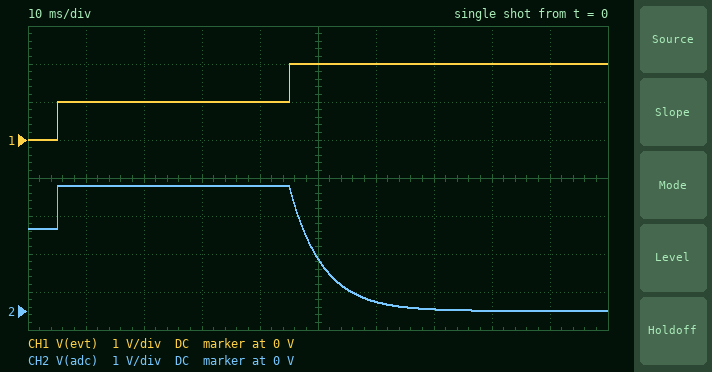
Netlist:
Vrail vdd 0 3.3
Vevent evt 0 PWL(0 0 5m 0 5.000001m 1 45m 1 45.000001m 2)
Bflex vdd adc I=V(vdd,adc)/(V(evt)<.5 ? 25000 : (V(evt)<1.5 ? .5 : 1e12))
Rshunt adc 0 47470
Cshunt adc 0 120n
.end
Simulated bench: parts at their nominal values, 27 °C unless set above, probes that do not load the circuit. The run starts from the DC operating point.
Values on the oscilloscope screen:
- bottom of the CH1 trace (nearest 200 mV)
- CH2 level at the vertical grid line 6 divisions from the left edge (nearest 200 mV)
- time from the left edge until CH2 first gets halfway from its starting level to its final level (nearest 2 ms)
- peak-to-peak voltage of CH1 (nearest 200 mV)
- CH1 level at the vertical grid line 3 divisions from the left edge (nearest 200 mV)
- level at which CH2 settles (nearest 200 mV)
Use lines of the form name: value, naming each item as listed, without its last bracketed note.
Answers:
bottom of the CH1 trace: 0 V
CH2 level at the vertical grid line 6 divisions from the left edge: 200 mV
time from the left edge until CH2 first gets halfway from its starting level to its final level: 52 ms
peak-to-peak voltage of CH1: 2.0 V
CH1 level at the vertical grid line 3 divisions from the left edge: 1.0 V
level at which CH2 settles: 0 V
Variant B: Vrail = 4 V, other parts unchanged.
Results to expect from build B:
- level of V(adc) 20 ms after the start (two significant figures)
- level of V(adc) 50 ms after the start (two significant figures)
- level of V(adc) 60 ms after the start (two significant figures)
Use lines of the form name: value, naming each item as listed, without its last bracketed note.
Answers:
level of V(adc) 20 ms after the start: 4.0 V
level of V(adc) 50 ms after the start: 1.7 V
level of V(adc) 60 ms after the start: 290 mV
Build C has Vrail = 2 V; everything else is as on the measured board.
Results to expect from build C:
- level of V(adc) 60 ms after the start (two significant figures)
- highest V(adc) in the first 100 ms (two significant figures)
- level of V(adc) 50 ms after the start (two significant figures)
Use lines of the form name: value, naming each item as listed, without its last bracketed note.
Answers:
level of V(adc) 60 ms after the start: 140 mV
highest V(adc) in the first 100 ms: 2.0 V
level of V(adc) 50 ms after the start: 830 mV
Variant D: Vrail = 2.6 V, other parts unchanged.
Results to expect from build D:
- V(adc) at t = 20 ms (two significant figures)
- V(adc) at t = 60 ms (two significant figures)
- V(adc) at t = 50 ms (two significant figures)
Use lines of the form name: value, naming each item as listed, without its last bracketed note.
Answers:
V(adc) at t = 20 ms: 2.6 V
V(adc) at t = 60 ms: 190 mV
V(adc) at t = 50 ms: 1.1 V
